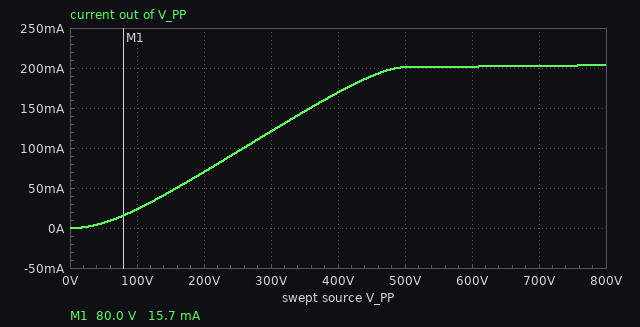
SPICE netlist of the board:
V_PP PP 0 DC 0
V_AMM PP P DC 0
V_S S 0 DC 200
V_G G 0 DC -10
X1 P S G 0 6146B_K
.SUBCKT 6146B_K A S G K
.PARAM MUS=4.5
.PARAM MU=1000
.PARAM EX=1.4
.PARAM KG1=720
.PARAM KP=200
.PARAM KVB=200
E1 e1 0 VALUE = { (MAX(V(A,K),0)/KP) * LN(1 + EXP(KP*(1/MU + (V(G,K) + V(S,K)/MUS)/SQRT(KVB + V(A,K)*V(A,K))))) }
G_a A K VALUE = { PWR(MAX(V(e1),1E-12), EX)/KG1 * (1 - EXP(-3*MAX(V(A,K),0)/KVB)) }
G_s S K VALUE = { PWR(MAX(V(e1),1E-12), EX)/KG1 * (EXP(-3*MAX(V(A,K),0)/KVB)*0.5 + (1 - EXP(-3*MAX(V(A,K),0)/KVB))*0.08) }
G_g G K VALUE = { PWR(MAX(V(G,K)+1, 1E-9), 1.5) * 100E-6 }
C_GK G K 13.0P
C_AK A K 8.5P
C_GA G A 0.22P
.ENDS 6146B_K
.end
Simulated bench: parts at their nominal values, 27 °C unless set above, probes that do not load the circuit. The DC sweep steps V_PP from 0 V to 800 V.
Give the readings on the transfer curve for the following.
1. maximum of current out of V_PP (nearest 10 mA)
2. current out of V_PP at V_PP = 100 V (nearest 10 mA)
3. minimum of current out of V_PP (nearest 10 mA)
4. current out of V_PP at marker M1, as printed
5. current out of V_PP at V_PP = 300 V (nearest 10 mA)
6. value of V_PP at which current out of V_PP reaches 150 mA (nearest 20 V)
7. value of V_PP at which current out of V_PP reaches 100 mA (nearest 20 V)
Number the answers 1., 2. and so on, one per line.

1. 200 mA
2. 20 mA
3. 0 A
4. 15.7 mA
5. 120 mA
6. 360 V
7. 260 V
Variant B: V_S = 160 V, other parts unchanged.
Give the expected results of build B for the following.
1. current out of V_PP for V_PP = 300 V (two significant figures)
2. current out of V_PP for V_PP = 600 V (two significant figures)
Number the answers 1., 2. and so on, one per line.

1. 110 mA
2. 130 mA
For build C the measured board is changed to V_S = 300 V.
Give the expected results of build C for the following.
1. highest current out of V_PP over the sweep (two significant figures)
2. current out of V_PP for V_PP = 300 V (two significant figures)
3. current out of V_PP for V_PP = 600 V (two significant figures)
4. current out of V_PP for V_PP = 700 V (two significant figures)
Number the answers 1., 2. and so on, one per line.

1. 400 mA
2. 130 mA
3. 310 mA
4. 360 mA
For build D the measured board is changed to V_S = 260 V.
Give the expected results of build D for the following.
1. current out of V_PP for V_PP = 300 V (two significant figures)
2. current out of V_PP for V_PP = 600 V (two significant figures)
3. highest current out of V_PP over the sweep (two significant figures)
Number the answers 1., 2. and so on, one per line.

1. 130 mA
2. 290 mA
3. 320 mA
